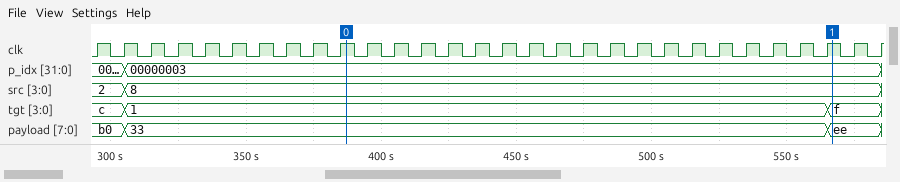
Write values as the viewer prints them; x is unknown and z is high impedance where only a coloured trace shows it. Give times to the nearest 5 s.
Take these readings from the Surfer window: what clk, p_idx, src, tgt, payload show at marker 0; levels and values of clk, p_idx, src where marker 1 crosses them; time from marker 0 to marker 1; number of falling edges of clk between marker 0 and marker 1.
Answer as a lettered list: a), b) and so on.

a) clk=1, p_idx=00000003, src=8, tgt=1, payload=33
b) clk=1, p_idx=00000003, src=8
c) 180 s
d) 18
